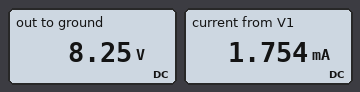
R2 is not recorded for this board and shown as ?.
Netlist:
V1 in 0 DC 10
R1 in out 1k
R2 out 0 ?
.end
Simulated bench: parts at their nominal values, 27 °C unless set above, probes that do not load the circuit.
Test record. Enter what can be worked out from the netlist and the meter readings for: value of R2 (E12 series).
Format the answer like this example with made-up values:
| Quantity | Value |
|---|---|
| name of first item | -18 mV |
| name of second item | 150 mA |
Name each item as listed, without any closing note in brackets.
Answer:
| Quantity | Value |
|---|---|
| value of R2 | 4.7 kΩ |
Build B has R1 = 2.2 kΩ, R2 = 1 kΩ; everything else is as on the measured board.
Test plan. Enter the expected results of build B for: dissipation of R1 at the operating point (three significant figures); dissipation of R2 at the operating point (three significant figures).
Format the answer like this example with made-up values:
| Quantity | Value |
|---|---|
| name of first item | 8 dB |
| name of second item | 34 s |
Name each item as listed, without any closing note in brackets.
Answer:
| Quantity | Value |
|---|---|
| dissipation of R1 at the operating point | 21.5 mW |
| dissipation of R2 at the operating point | 9.77 mW |
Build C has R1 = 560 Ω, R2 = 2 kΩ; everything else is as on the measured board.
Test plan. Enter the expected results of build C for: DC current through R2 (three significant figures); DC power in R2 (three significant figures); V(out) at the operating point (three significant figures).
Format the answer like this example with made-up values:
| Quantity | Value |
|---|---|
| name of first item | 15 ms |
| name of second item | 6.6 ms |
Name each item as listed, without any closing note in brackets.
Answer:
| Quantity | Value |
|---|---|
| DC current through R2 | 3.91 mA |
| DC power in R2 | 30.5 mW |
| V(out) at the operating point | 7.81 V |
